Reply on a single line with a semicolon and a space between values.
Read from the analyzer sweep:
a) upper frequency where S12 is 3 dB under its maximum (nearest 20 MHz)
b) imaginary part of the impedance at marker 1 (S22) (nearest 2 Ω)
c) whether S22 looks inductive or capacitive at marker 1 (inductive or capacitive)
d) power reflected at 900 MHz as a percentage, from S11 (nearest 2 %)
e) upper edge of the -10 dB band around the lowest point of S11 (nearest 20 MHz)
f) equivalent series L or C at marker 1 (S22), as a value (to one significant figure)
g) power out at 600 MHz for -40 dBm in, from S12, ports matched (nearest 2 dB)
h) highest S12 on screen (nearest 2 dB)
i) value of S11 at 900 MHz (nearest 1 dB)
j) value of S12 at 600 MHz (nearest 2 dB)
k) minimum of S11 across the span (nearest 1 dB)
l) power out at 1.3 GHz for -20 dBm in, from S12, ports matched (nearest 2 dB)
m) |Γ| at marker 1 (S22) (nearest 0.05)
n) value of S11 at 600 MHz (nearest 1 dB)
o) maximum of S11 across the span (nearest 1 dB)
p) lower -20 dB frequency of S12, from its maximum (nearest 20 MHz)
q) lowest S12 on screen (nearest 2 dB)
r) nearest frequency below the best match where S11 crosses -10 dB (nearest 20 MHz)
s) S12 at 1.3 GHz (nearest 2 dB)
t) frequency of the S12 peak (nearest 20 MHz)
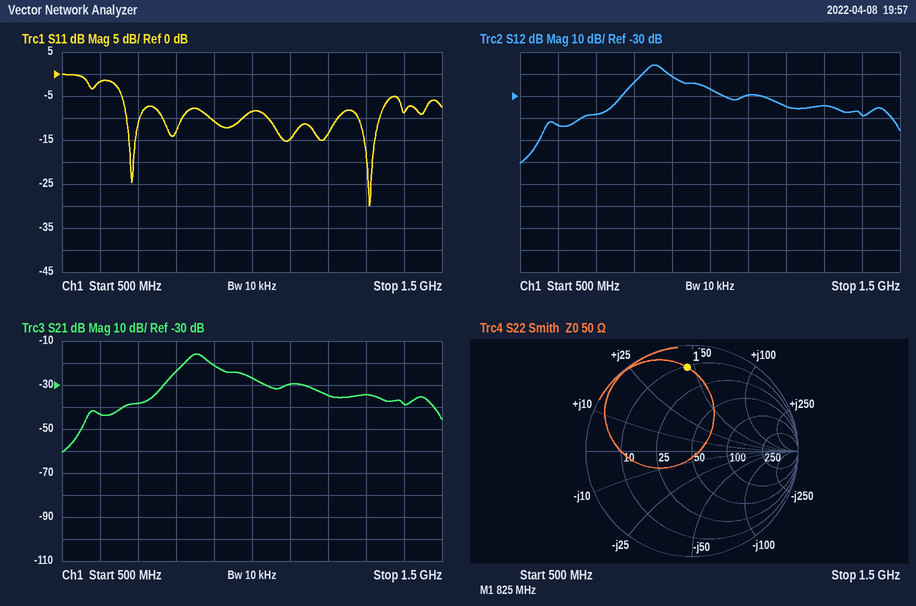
880 MHz; +46 Ω; inductive; 8 %; 1.34 GHz; 9 nH; -84 dBm; -16 dB; -11 dB; -44 dB; -30 dB; -54 dBm; 0.80; -2 dB; 0 dB; 740 MHz; -60 dB; 1.28 GHz; -34 dB; 860 MHz
